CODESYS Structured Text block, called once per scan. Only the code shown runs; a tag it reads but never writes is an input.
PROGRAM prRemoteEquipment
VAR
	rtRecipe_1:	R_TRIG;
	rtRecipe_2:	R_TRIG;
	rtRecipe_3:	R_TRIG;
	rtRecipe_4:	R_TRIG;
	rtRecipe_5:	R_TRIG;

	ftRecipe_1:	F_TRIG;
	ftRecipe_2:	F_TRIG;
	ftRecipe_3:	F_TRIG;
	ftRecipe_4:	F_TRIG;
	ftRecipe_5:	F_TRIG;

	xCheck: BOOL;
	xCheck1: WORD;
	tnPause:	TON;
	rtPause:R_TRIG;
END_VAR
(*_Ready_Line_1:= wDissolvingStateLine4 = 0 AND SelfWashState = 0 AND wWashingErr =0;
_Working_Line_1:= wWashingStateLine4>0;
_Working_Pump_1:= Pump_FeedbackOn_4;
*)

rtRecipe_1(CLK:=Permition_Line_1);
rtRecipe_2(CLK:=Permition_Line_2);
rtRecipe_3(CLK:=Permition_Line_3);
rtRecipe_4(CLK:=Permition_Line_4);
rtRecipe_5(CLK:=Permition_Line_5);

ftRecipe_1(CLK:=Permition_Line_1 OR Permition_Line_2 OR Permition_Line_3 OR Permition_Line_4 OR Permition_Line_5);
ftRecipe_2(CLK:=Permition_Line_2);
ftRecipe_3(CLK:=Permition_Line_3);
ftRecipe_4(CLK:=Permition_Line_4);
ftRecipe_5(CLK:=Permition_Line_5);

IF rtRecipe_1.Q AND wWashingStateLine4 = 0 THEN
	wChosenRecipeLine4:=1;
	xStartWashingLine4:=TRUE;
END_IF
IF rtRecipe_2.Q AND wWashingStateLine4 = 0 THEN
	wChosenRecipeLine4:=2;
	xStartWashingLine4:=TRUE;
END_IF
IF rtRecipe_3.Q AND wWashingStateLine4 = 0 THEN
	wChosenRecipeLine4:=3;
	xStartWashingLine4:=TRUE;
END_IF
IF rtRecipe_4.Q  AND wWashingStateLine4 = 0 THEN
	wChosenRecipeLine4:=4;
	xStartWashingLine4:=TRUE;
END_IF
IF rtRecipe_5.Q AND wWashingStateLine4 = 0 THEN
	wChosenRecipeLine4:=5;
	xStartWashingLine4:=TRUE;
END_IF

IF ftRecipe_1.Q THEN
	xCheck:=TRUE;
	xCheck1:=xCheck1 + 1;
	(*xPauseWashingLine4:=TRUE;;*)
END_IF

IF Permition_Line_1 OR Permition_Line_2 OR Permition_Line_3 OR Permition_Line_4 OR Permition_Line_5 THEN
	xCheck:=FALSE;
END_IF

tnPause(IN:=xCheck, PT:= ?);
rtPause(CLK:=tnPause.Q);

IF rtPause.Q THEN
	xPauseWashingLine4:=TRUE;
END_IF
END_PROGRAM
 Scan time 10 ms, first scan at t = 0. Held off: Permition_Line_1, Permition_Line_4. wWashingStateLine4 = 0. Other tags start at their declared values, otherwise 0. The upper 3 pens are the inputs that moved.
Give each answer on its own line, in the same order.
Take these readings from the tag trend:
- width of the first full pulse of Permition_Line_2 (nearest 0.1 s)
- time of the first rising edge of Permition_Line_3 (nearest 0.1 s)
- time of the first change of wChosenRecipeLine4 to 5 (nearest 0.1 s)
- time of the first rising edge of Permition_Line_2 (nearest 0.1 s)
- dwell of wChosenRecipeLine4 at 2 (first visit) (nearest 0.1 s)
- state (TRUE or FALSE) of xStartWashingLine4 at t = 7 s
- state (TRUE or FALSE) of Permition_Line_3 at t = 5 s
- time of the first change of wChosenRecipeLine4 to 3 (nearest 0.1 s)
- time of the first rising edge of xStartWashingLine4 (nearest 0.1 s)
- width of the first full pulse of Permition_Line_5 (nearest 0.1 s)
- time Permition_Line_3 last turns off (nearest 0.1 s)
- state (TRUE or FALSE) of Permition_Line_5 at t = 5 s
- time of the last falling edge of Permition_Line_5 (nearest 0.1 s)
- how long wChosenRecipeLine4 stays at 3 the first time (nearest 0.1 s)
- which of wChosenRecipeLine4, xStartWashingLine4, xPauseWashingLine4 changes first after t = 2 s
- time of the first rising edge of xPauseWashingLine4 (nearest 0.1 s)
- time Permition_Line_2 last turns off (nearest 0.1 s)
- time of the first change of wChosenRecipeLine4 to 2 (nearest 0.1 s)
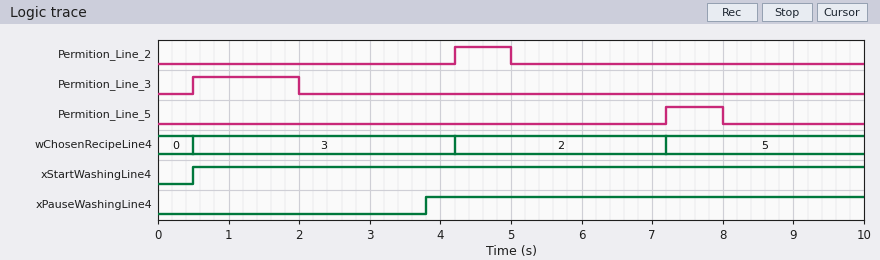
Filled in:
0.8 s
0.5 s
7.2 s
4.2 s
3.0 s
TRUE
FALSE
0.5 s
0.5 s
0.8 s
2.0 s
FALSE
8.0 s
3.7 s
xPauseWashingLine4
3.8 s
5.0 s
4.2 s
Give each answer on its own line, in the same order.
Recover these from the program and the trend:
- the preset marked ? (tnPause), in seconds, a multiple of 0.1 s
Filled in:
1.8 s
